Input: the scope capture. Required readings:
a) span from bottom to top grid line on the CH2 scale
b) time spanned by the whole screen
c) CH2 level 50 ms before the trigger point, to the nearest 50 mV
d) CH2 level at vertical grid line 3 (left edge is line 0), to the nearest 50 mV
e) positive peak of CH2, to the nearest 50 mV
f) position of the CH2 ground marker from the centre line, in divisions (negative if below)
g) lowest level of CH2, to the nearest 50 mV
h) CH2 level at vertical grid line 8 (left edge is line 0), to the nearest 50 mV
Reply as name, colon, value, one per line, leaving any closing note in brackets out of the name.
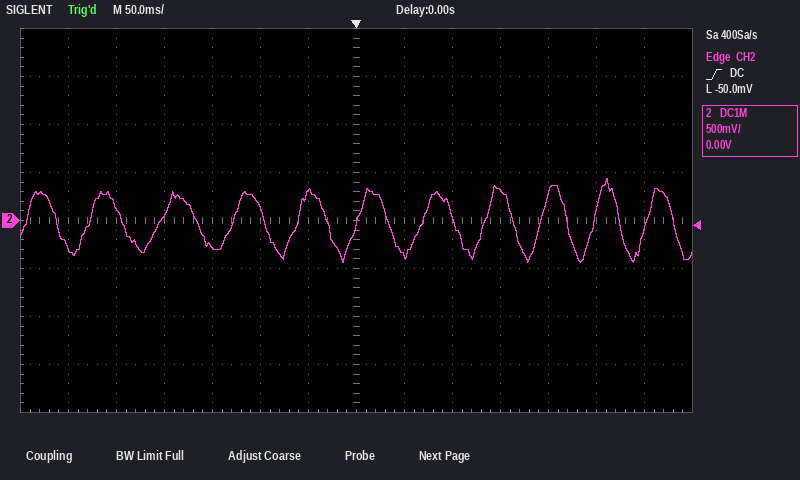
span from bottom to top grid line on the CH2 scale: 4 V
time spanned by the whole screen: 700 ms
CH2 level 50 ms before the trigger point, to the nearest 50 mV: 300 mV
CH2 level at vertical grid line 3 (left edge is line 0), to the nearest 50 mV: 50 mV
positive peak of CH2, to the nearest 50 mV: 450 mV
position of the CH2 ground marker from the centre line, in divisions: 0.0 div
lowest level of CH2, to the nearest 50 mV: -450 mV
CH2 level at vertical grid line 8 (left edge is line 0), to the nearest 50 mV: -350 mV
